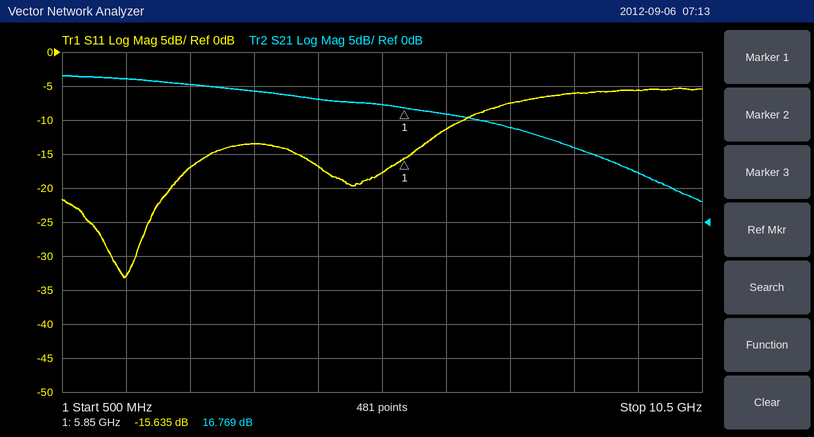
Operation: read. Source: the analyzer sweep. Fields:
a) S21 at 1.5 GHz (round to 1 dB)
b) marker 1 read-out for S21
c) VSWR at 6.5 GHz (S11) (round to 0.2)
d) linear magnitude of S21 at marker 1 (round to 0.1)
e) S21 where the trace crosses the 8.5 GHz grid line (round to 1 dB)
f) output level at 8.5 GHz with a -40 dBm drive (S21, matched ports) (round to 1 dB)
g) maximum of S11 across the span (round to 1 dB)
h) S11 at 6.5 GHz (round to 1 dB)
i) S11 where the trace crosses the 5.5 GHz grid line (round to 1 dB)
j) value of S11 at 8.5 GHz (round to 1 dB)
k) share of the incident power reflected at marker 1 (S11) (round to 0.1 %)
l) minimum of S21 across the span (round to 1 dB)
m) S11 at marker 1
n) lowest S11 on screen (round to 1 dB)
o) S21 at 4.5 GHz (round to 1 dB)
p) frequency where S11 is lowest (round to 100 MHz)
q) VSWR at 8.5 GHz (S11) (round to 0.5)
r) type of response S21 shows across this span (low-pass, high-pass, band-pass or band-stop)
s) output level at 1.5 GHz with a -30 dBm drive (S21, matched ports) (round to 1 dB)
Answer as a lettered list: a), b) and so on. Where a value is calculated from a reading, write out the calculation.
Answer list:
a) 21 dB
b) 16.769 dB
c) |Γ| = 10^(-11/20) = 0.2818; VSWR = (1 + 0.2818)/(1 − 0.2818) ≈ 1.8
d) 10^(16.769/20) ≈ 6.9
e) 11 dB
f) -40 dBm + (11 dB) = -29 dBm
g) -5 dB
h) -11 dB
i) -18 dB
j) -6 dB
k) 10^(-15.635/10) ≈ 2.7 %
l) 3 dB
m) -15.635 dB
n) -33 dB
o) 18 dB
p) 1.5 GHz
q) |Γ| = 10^(-6/20) = 0.5012; VSWR = (1 + 0.5012)/(1 − 0.5012) ≈ 3.0
r) low-pass
s) -30 dBm + (21 dB) = -9 dBm
